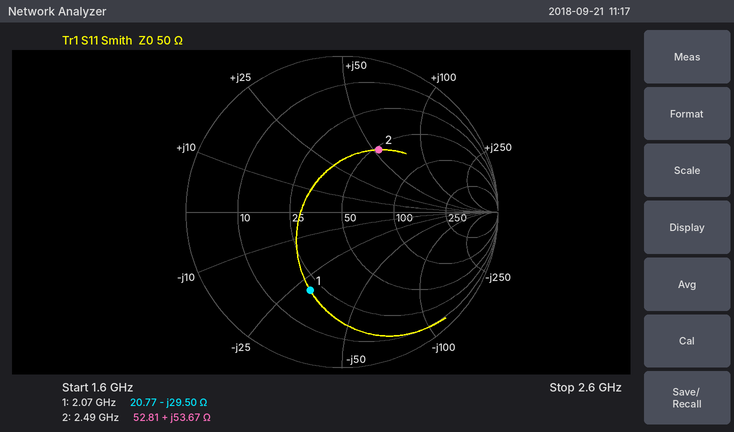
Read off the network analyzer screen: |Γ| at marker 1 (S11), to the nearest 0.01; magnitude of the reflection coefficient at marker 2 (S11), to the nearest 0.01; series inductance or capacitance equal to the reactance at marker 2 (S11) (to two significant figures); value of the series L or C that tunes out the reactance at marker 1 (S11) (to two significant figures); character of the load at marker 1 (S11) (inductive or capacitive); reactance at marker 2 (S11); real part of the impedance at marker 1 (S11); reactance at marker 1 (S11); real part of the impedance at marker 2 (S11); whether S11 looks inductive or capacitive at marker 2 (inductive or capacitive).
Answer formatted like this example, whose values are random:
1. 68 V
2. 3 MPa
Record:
1. 0.54
2. 0.46
3. 3.4 nH
4. 2.3 nH
5. capacitive
6. +53.67 Ω
7. 20.77 Ω
8. -29.50 Ω
9. 52.81 Ω
10. inductive
